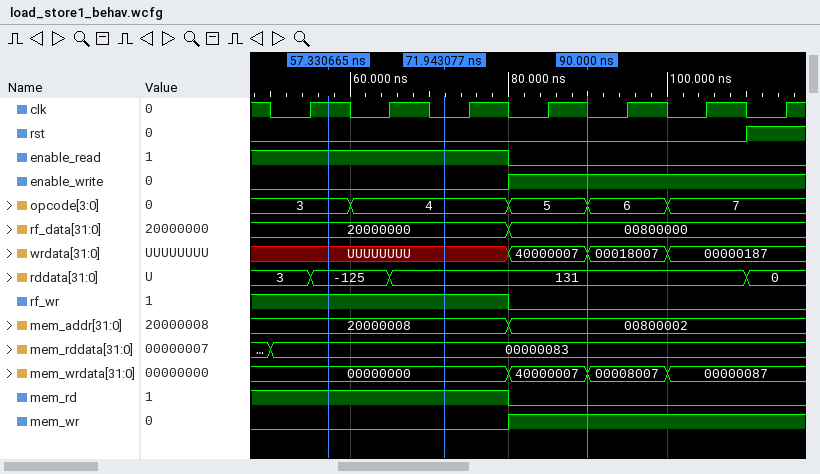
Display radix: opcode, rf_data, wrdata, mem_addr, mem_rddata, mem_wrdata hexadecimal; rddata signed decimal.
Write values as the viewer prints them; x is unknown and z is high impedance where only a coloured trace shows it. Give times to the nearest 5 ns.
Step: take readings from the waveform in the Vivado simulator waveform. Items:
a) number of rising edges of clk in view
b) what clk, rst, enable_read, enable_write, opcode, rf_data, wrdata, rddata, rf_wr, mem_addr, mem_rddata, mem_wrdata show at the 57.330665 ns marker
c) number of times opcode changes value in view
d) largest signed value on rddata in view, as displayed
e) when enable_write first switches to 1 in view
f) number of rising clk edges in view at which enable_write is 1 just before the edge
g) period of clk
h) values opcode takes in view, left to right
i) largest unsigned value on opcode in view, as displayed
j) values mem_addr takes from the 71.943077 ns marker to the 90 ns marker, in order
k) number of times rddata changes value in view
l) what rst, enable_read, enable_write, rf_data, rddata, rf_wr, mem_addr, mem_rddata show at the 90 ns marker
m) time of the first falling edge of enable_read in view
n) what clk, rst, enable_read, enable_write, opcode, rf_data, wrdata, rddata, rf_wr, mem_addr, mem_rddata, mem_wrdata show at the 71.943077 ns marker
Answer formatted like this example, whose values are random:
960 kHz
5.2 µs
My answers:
7
clk=1, rst=0, enable_read=1, enable_write=0, opcode=3, rf_data=20000000, wrdata=UUUUUUUU, rddata=-125, rf_wr=1, mem_addr=20000008, mem_rddata=00000083, mem_wrdata=00000000
4
131
80 ns
4
10 ns
3, 4, 5, 6, 7
7
20000008, 00800002
3
rst=0, enable_read=0, enable_write=1, rf_data=00800000, rddata=131, rf_wr=0, mem_addr=00800002, mem_rddata=00000083
80 ns
clk=0, rst=0, enable_read=1, enable_write=0, opcode=4, rf_data=20000000, wrdata=UUUUUUUU, rddata=131, rf_wr=1, mem_addr=20000008, mem_rddata=00000083, mem_wrdata=00000000
